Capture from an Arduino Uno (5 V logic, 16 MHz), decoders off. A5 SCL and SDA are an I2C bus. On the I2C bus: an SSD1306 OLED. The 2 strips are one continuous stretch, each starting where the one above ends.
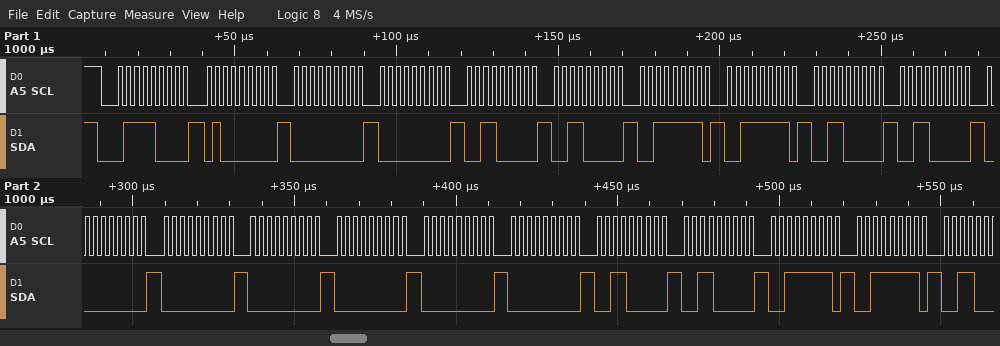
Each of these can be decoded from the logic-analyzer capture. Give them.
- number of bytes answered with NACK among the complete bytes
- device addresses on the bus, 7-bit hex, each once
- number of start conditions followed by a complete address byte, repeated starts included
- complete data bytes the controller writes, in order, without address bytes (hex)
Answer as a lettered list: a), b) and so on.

a) 0
b) 0x3C
c) 1
d) 40 00 00 30 30 3F 3F 30 30 00 00 00 00 00 00 30 30 3F 3F
